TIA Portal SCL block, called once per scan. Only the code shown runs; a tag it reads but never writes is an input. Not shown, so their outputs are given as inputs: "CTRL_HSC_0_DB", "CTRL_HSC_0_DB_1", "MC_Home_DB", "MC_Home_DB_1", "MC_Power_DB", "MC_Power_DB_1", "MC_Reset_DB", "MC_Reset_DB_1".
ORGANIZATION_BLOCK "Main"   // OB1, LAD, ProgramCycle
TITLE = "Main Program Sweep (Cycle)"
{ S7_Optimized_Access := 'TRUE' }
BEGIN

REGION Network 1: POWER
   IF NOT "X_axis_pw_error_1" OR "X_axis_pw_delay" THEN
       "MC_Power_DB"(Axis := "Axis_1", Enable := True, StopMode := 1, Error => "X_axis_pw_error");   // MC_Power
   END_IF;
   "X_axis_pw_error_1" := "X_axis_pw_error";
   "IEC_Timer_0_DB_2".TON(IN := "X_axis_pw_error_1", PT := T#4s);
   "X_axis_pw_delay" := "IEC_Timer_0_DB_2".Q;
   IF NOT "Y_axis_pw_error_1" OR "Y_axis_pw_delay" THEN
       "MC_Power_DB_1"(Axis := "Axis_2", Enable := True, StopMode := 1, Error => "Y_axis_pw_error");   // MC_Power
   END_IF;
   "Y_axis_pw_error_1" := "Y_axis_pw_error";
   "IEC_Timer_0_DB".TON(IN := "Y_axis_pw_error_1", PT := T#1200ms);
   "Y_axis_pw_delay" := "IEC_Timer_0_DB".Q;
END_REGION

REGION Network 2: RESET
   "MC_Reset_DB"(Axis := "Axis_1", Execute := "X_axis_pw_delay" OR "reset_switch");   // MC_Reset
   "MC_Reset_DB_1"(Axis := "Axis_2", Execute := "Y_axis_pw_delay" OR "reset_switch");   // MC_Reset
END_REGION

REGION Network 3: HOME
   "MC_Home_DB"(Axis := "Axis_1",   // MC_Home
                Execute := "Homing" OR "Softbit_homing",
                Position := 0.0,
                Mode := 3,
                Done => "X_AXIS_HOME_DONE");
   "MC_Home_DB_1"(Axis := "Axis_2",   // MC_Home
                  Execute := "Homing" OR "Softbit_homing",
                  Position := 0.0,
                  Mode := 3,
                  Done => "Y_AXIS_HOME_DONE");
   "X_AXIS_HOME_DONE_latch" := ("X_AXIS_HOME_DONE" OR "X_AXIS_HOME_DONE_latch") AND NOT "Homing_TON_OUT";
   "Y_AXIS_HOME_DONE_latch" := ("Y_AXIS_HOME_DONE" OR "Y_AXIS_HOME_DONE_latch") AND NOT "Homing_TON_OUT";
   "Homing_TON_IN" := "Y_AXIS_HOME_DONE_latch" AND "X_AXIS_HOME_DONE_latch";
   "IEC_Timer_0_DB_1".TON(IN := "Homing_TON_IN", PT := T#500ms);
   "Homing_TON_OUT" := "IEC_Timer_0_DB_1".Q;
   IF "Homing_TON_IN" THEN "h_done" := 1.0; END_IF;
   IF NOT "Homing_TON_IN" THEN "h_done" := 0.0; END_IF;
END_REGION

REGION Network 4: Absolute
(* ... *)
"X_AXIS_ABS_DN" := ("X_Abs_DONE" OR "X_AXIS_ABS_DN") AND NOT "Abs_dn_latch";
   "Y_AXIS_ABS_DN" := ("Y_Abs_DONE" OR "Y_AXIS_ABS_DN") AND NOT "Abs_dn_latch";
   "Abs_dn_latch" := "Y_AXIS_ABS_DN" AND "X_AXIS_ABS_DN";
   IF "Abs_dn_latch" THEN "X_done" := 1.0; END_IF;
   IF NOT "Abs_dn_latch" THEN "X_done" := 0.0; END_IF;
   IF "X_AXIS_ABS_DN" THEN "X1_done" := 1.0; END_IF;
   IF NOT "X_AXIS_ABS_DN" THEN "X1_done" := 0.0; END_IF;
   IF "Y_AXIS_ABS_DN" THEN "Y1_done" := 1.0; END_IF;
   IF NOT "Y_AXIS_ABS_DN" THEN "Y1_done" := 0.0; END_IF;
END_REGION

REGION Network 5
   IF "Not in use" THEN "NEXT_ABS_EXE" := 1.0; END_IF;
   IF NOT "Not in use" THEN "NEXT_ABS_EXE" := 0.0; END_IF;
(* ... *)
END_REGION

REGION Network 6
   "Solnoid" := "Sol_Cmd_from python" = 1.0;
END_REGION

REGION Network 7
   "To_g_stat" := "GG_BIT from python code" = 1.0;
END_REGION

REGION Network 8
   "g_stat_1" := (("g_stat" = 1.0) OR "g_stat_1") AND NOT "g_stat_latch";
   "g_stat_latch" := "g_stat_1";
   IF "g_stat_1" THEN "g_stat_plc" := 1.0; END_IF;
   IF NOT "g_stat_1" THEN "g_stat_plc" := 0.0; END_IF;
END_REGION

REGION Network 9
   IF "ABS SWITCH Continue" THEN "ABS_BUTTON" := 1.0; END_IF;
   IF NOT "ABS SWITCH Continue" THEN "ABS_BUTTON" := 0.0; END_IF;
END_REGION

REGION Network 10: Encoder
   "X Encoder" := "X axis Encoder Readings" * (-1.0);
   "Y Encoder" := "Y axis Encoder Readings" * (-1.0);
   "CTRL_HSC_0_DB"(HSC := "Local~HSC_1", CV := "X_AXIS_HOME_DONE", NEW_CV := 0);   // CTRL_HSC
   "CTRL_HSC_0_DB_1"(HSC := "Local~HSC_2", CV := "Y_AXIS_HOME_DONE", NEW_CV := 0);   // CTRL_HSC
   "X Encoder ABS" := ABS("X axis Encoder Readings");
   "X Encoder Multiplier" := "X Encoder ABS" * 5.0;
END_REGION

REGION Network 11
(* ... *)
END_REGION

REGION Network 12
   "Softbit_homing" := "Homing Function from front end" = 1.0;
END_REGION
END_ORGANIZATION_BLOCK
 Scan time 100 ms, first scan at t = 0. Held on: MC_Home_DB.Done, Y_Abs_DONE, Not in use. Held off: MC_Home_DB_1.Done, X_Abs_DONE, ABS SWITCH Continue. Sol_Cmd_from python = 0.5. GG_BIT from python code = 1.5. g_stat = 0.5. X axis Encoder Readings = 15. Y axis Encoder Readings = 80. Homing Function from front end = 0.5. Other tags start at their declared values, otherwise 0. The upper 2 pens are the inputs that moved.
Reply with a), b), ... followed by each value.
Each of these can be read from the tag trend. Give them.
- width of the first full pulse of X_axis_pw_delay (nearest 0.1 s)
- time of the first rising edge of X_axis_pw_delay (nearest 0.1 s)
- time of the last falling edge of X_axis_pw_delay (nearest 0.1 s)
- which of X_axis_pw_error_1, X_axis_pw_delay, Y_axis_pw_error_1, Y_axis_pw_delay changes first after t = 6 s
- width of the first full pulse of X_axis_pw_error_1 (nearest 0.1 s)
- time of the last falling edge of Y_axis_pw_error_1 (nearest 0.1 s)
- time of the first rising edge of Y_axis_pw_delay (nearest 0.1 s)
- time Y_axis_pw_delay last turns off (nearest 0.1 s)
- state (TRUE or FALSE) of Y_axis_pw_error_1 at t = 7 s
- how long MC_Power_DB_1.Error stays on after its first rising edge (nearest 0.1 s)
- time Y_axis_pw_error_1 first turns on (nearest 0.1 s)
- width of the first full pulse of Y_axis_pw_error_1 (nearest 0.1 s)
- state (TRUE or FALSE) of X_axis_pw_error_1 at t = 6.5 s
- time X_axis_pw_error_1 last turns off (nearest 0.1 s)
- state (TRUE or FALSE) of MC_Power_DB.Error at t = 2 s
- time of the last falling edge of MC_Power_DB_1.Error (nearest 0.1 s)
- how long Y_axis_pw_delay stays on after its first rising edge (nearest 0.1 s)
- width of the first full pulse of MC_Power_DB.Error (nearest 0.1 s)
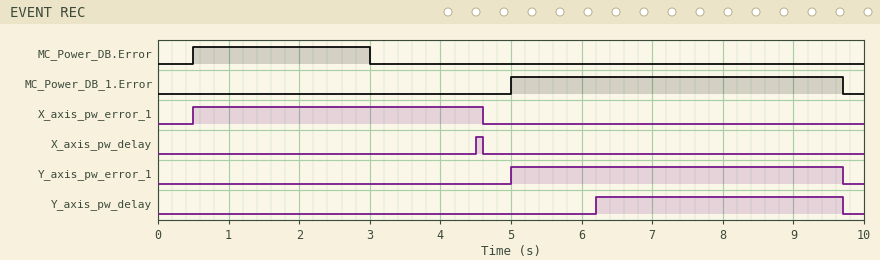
a) 0.1 s
b) 4.5 s
c) 4.6 s
d) Y_axis_pw_delay
e) 4.1 s
f) 9.7 s
g) 6.2 s
h) 9.7 s
i) TRUE
j) 4.7 s
k) 5.0 s
l) 4.7 s
m) FALSE
n) 4.6 s
o) TRUE
p) 9.7 s
q) 3.5 s
r) 2.5 s
